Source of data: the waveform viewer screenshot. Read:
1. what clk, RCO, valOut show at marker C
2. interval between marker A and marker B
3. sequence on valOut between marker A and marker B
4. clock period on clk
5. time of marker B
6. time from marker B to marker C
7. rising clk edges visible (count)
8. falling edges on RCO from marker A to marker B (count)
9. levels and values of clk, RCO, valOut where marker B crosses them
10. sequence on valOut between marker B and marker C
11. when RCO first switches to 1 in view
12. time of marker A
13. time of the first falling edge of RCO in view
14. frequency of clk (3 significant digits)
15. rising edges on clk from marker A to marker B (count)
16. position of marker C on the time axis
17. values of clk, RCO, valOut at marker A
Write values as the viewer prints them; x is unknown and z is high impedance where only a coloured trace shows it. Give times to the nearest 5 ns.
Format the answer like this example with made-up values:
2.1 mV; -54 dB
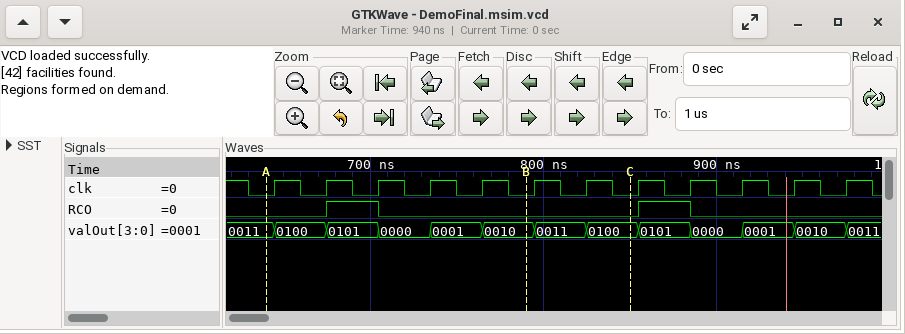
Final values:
clk=0, RCO=0, valOut=0100; 150 ns; 0011, 0100, 0101, 0000, 0001, 0010; 30 ns; 790 ns; 60 ns; 12; 1; clk=0, RCO=0, valOut=0010; 0010, 0011, 0100; 675 ns; 640 ns; 705 ns; 33.3 MHz; 5; 850 ns; clk=0, RCO=0, valOut=0011
